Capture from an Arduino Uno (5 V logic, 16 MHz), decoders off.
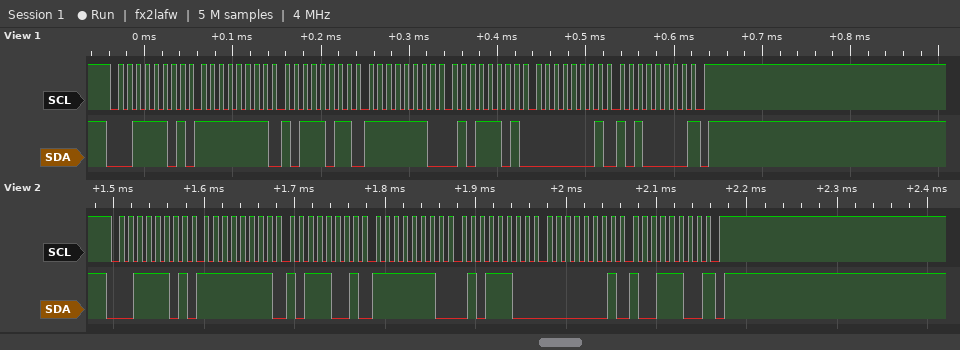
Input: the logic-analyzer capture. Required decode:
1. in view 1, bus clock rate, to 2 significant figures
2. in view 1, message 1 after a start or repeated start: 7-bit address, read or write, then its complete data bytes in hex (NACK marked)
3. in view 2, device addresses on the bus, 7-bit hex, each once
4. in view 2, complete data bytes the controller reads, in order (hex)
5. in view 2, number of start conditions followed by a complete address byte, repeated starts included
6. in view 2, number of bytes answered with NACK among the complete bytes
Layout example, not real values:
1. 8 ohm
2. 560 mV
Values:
1. 100 kHz
2. 0x1E read: FF BB FE 5D 01 A0 NACK
3. 0x1E
4. FF B9 FE 5C 01 9C
5. 1
6. 1
